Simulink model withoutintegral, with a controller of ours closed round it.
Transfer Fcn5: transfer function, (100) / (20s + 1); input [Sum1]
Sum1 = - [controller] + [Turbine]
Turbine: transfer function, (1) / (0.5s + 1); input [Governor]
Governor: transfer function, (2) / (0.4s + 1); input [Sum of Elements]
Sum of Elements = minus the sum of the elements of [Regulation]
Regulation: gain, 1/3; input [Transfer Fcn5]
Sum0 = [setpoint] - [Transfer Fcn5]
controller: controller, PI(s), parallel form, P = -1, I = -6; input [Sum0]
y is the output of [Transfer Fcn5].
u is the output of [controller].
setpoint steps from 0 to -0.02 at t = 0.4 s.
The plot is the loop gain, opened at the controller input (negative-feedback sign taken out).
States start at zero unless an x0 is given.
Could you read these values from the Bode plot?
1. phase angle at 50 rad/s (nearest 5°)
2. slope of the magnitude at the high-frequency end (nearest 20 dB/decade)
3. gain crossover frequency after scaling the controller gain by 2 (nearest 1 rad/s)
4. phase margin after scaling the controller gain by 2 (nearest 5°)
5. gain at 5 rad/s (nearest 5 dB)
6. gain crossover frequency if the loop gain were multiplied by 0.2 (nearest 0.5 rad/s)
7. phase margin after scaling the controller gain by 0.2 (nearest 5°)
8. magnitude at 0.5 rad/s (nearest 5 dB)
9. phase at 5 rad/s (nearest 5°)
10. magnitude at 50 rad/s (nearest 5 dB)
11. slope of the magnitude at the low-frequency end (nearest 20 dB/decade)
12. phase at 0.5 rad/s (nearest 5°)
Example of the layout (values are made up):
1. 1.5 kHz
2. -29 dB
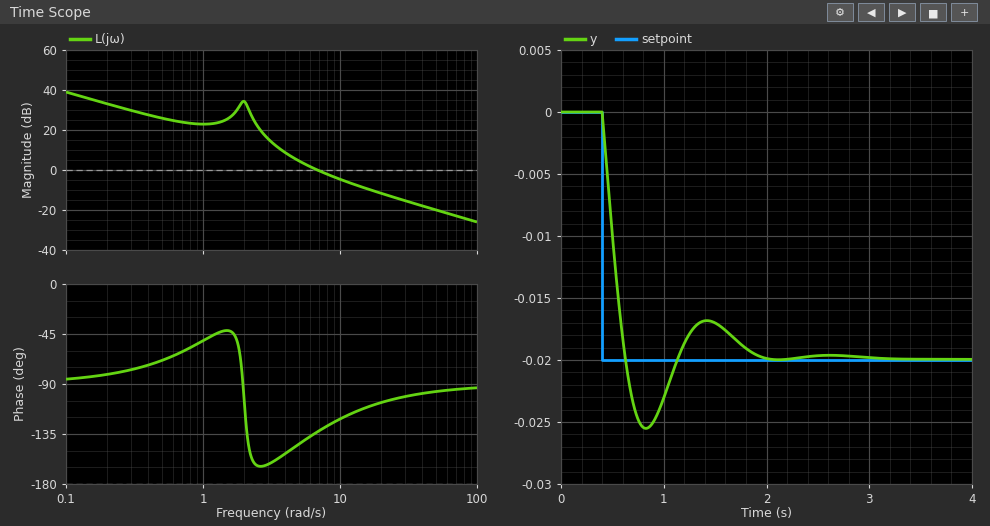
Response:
1. -95°
2. -20 dB/decade
3. 11 rad/s
4. 60°
5. 5 dB
6. 3.0 rad/s
7. 20°
8. 25 dB
9. -145°
10. -20 dB
11. -20 dB/decade
12. -70°
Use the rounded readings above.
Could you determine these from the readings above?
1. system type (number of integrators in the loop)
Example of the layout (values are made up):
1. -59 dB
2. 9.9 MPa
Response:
1. 1
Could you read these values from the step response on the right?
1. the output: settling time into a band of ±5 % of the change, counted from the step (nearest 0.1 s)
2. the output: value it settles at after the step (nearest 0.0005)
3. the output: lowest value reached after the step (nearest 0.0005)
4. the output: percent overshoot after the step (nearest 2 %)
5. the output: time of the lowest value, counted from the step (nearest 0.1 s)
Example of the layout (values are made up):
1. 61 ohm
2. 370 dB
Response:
1. 1.4 s
2. -0.0200
3. -0.0255
4. 28 %
5. 0.4 s
